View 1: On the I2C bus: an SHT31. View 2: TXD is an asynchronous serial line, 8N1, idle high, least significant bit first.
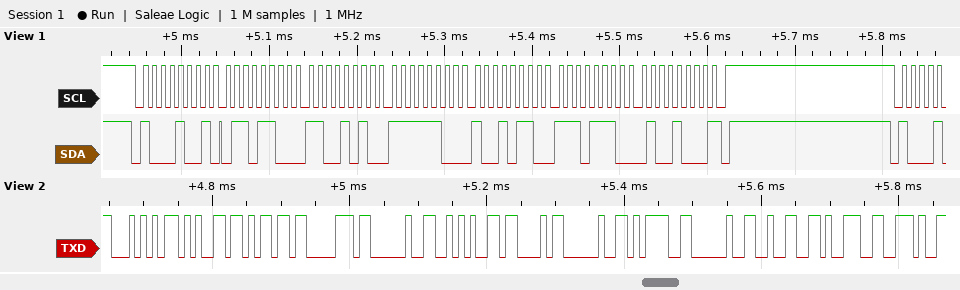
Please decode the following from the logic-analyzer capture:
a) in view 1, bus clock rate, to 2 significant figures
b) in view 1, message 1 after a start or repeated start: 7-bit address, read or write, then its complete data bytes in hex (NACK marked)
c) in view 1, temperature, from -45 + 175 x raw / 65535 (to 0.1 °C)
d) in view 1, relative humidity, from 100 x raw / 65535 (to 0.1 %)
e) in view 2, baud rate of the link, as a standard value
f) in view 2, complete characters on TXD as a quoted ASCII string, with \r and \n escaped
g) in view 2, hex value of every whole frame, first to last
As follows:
100 kHz
0x44 read: 6C CA FC 96 EE 48 NACK
29.4 °C
59.0 %
115200 baud
"Temp *C = 29."
54 65 6D 70 20 2A 43 20 3D 20 32 39 2E
